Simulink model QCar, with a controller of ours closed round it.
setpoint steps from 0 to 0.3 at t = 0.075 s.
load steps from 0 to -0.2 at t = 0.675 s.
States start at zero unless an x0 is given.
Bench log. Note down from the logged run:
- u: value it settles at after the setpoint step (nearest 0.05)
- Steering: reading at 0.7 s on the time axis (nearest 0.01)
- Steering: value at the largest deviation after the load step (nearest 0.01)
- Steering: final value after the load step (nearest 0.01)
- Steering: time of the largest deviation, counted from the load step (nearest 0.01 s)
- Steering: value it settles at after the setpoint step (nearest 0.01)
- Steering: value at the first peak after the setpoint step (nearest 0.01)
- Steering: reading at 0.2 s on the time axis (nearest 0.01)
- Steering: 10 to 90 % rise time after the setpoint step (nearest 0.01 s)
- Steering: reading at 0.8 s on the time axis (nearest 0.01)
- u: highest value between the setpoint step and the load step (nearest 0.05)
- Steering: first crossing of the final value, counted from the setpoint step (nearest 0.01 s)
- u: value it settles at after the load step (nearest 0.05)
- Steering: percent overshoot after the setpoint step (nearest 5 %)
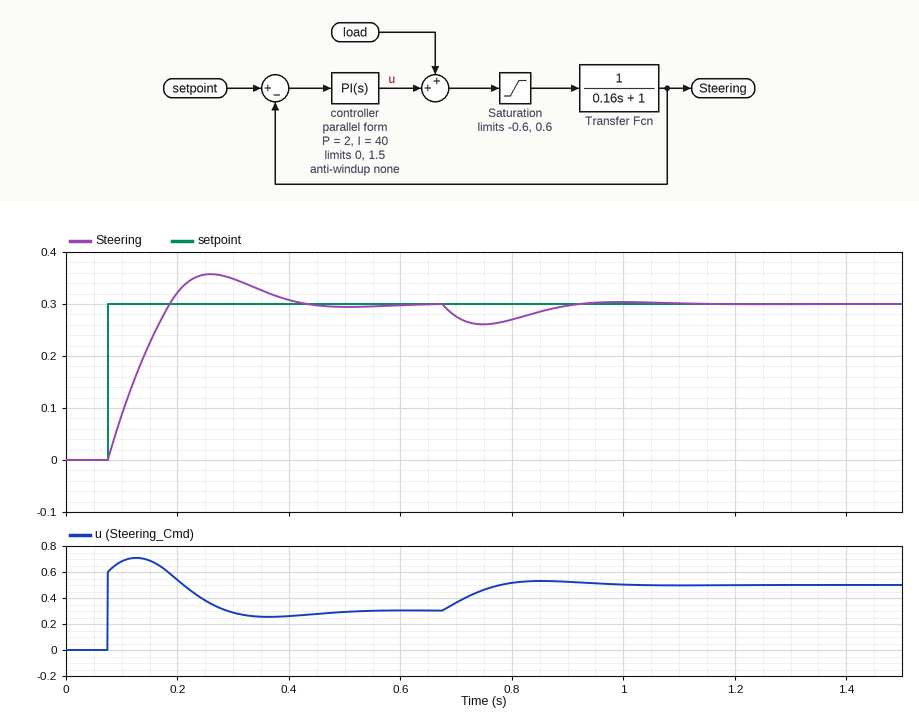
0.30
0.28
0.26
0.30
0.07 s
0.30
0.36
0.32
0.09 s
0.27
0.70
0.11 s
0.50
20 %
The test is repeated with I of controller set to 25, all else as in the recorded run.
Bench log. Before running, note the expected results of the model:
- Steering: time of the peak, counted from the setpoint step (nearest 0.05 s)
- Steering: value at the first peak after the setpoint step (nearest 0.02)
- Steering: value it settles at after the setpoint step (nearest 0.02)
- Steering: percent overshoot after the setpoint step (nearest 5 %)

0.25 s
0.32
0.30
10 %
